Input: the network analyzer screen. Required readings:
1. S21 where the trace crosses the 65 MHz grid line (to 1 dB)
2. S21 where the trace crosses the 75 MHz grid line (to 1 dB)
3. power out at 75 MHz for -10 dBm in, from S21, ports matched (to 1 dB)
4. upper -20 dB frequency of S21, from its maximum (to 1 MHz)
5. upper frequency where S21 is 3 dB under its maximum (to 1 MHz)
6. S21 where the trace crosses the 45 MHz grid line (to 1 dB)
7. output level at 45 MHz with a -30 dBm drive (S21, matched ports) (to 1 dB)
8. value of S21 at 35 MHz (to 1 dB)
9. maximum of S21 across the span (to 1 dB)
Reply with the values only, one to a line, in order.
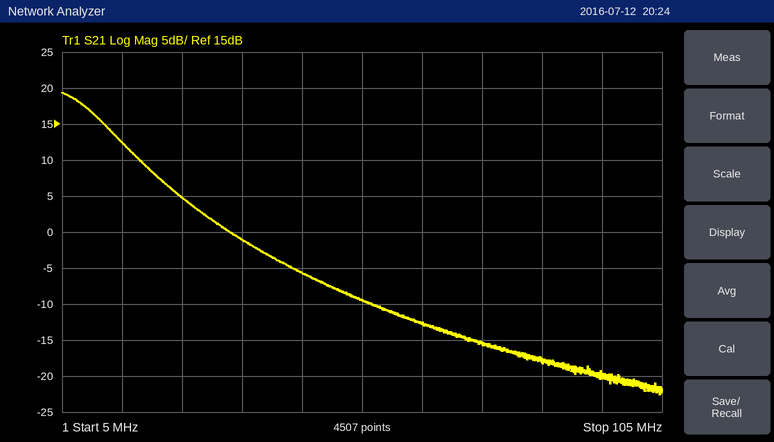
-13 dB
-15 dB
-25 dBm
34 MHz
10 MHz
-6 dB
-36 dBm
-1 dB
19 dB
